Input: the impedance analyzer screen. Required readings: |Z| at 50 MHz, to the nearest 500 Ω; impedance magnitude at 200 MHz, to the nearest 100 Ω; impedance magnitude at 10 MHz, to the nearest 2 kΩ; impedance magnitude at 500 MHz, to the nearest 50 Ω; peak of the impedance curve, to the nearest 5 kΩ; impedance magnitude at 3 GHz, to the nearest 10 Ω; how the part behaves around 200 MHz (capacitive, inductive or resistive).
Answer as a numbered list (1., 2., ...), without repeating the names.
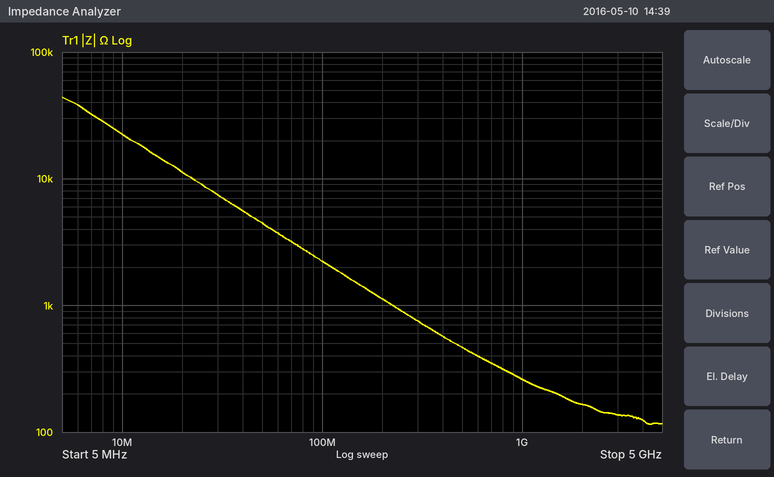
1. 4.5 kΩ
2. 1.1 kΩ
3. 22 kΩ
4. 450 Ω
5. 45 kΩ
6. 140 Ω
7. capacitive
